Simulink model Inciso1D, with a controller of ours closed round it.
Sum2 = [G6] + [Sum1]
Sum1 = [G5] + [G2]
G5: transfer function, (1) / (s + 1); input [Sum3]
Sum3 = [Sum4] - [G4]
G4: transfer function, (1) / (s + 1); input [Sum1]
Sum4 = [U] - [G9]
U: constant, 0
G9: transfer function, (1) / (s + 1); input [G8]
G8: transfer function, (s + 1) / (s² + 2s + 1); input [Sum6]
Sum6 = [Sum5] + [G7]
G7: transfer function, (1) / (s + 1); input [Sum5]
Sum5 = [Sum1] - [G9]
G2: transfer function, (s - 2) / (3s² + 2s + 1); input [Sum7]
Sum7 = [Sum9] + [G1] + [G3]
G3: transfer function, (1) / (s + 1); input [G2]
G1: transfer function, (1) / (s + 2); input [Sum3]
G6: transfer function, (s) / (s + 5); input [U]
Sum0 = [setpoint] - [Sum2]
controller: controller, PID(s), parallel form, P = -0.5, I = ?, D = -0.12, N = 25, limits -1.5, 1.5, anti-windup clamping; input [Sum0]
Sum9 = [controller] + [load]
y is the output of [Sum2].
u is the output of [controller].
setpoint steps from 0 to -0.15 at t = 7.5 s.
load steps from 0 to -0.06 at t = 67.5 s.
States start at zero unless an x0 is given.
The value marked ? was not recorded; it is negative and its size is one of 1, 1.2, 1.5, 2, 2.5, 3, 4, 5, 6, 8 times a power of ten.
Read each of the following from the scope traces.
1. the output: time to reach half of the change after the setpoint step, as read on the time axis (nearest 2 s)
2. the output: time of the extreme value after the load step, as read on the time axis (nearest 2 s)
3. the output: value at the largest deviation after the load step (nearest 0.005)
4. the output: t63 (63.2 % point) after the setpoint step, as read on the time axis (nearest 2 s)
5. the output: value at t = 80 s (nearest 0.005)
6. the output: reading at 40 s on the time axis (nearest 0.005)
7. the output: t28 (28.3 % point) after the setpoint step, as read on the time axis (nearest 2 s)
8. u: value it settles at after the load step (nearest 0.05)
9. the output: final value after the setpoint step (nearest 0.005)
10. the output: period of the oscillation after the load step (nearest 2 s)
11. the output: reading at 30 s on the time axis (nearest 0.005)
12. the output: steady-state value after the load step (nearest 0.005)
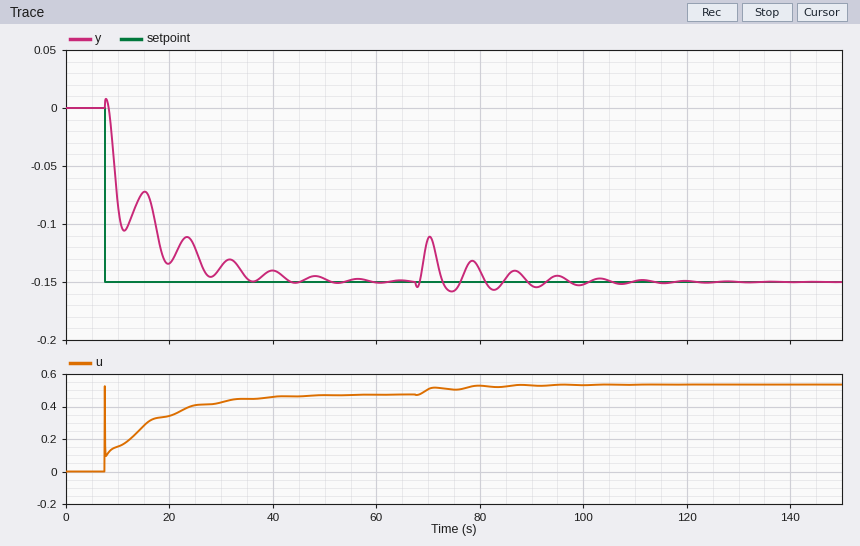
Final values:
10 s
70 s
-0.110
10 s
-0.140
-0.140
10 s
0.55
-0.150
8 s
-0.135
-0.150
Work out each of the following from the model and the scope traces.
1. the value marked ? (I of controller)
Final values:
-0.4
